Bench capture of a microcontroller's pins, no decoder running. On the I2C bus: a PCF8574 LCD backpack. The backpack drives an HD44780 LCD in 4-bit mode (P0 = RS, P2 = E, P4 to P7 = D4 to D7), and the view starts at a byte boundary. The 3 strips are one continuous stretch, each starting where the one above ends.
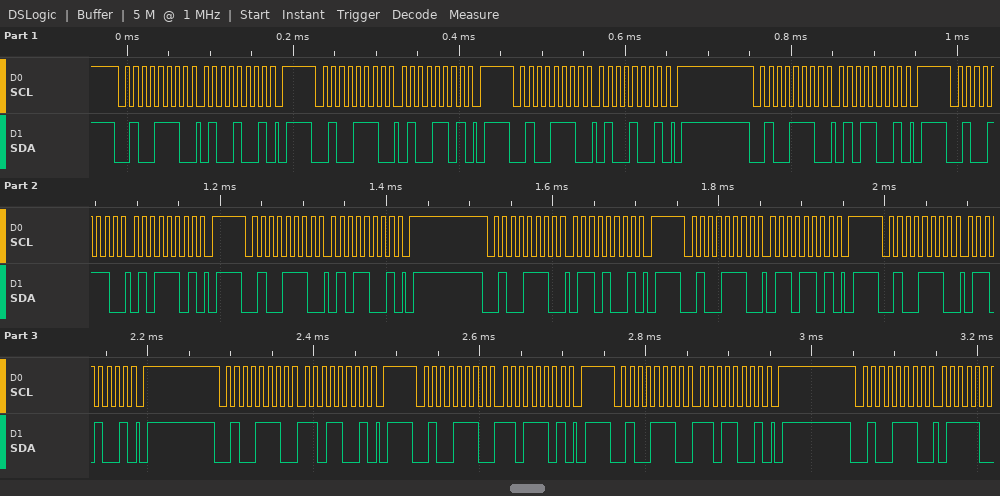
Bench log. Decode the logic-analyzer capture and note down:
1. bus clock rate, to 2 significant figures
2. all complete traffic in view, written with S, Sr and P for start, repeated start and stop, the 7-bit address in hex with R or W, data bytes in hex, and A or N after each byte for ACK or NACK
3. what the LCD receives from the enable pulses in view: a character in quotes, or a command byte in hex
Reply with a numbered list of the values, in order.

1. 100 kHz
2. S 27W A 49 A P S 27W A 4D A P S 27W A 49 A P S 27W A 59 A P S 27W A 5D A P S 27W A 59 A P S 27W A 69 A P S 27W A 6D A P S 27W A 69 A P S 27W A D9 A P S 27W A DD A P S 27W A D9 A P S 27W A
3. 'E' 'm'
